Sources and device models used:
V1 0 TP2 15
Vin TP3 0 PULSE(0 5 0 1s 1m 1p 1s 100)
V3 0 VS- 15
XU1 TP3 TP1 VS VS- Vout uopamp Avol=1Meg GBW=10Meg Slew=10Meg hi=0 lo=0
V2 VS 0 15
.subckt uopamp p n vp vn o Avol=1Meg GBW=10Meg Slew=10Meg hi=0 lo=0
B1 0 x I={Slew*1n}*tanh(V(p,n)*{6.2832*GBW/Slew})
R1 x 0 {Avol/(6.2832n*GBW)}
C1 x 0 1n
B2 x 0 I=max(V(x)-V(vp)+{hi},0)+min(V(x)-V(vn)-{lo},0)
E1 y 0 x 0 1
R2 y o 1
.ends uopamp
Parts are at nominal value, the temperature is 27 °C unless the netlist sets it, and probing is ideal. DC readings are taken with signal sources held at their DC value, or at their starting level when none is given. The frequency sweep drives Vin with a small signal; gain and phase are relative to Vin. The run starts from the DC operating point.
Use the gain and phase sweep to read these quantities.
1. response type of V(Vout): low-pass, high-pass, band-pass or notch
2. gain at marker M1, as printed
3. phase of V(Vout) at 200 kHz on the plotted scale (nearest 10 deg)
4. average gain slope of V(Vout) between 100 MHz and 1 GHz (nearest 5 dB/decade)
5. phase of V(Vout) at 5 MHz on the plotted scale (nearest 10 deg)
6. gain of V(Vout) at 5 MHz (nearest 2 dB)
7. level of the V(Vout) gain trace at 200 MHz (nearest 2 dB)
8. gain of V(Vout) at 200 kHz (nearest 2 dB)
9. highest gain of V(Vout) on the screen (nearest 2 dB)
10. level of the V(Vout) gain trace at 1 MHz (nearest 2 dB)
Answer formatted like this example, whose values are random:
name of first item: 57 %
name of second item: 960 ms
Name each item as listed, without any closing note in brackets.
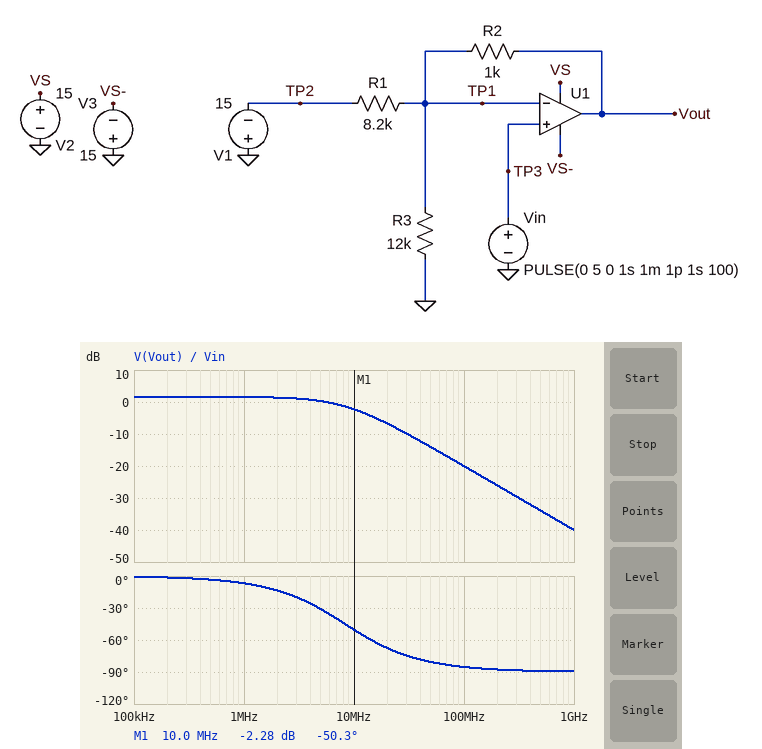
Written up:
response type of V(Vout): low-pass, high-pass, band-pass or notch: low-pass
gain at marker M1, as printed: -2.28 dB
phase of V(Vout) at 200 kHz on the plotted scale: 0 deg
average gain slope of V(Vout) between 100 MHz and 1 GHz: -20 dB/decade
phase of V(Vout) at 5 MHz on the plotted scale: -30 deg
gain of V(Vout) at 5 MHz: 0 dB
level of the V(Vout) gain trace at 200 MHz: -26 dB
gain of V(Vout) at 200 kHz: 2 dB
highest gain of V(Vout) on the screen: 2 dB
level of the V(Vout) gain trace at 1 MHz: 2 dB
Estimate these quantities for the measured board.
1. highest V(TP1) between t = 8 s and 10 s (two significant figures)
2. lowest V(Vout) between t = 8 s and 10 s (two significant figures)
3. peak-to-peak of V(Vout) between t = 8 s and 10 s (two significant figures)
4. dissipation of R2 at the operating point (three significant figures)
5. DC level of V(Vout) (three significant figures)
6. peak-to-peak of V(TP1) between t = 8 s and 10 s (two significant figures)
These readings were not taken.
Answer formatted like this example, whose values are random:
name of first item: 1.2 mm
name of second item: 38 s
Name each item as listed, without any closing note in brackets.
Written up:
highest V(TP1) between t = 8 s and 10 s: 5.0 V
lowest V(Vout) between t = 8 s and 10 s: 1.8 V
peak-to-peak of V(Vout) between t = 8 s and 10 s: 6.0 V
dissipation of R2 at the operating point: 3.35 mW
DC level of V(Vout): 1.83 V
peak-to-peak of V(TP1) between t = 8 s and 10 s: 5.0 V
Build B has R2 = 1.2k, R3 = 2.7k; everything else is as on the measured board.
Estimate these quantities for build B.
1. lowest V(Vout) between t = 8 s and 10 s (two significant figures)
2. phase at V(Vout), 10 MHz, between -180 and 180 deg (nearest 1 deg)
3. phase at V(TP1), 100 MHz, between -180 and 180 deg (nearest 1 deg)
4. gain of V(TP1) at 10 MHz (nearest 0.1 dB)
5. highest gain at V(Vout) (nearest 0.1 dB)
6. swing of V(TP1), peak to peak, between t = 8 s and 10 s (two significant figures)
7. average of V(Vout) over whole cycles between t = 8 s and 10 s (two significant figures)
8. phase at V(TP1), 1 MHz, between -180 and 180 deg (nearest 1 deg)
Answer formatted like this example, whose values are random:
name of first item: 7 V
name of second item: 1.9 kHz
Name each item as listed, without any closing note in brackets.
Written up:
lowest V(Vout) between t = 8 s and 10 s: 2.2 V
phase at V(Vout), 10 MHz, between -180 and 180 deg: -58 deg
phase at V(TP1), 100 MHz, between -180 and 180 deg: -86 deg
gain of V(TP1) at 10 MHz: -5.5 dB
highest gain at V(Vout): 4.0 dB
swing of V(TP1), peak to peak, between t = 8 s and 10 s: 5.0 V
average of V(Vout) over whole cycles between t = 8 s and 10 s: 6.2 V
phase at V(TP1), 1 MHz, between -180 and 180 deg: -9 deg
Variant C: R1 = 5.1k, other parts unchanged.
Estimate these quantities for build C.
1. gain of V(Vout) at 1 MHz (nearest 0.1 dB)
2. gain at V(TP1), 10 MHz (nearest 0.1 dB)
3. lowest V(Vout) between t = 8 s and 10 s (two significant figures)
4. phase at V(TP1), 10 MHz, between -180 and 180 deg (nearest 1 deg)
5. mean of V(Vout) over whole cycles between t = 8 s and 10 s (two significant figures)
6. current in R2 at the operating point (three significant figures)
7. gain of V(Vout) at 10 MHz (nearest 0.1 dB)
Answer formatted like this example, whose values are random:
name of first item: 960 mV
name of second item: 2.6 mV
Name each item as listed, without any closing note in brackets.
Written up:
gain of V(Vout) at 1 MHz: 2.1 dB
gain at V(TP1), 10 MHz: -4.2 dB
lowest V(Vout) between t = 8 s and 10 s: 2.9 V
phase at V(TP1), 10 MHz, between -180 and 180 deg: -52 deg
mean of V(Vout) over whole cycles between t = 8 s and 10 s: 6.1 V
current in R2 at the operating point: 2.94 mA
gain of V(Vout) at 10 MHz: -2.1 dB
